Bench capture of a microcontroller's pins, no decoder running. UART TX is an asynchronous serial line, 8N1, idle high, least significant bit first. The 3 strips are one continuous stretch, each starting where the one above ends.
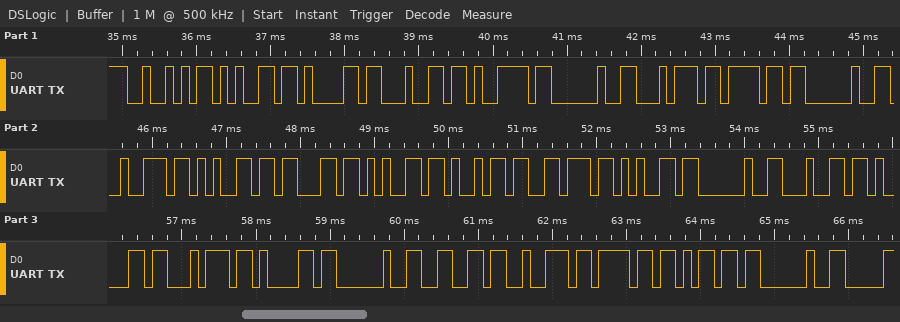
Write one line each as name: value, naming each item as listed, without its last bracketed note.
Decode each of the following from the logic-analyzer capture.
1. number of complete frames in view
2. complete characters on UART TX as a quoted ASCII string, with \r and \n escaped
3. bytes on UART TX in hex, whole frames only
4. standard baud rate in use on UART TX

number of complete frames in view: 27
complete characters on UART TX as a quoted ASCII string, with \r and \n escaped: "Ready to receive data from "
bytes on UART TX in hex, whole frames only: 52 65 61 64 79 20 74 6F 20 72 65 63 65 69 76 65 20 64 61 74 61 20 66 72 6F 6D 20
standard baud rate in use on UART TX: 9600 baud
